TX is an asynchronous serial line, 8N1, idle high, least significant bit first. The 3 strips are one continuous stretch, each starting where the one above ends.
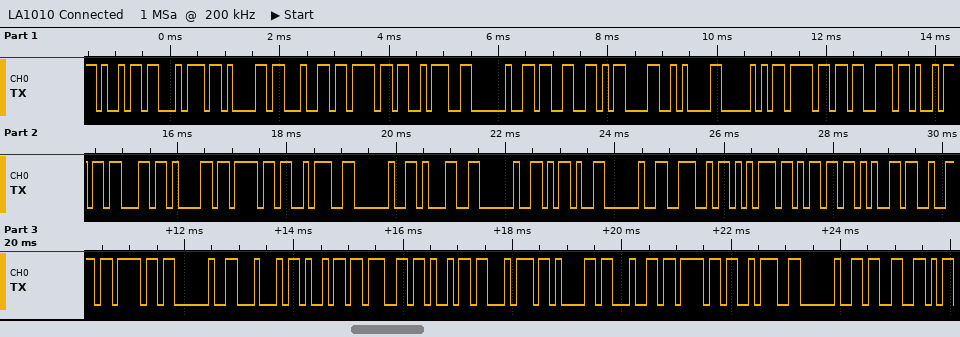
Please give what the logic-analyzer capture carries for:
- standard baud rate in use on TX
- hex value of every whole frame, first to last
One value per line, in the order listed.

9600 baud
0x69 0x74 0x61 0x64 0x6F 0x3A 0x20 0x33 0x0D 0x0A 0x50 0x6F 0x73 0x69 0x63 0x61 0x6F 0x3A 0x20 0x31 0x20 0x2D 0x20 0x4E 0x75 0x6D 0x65 0x72 0x6F 0x20 0x44 0x69 0x67 0x69 0x74 0x61 0x64 0x6F 0x3A 0x20 0x33
